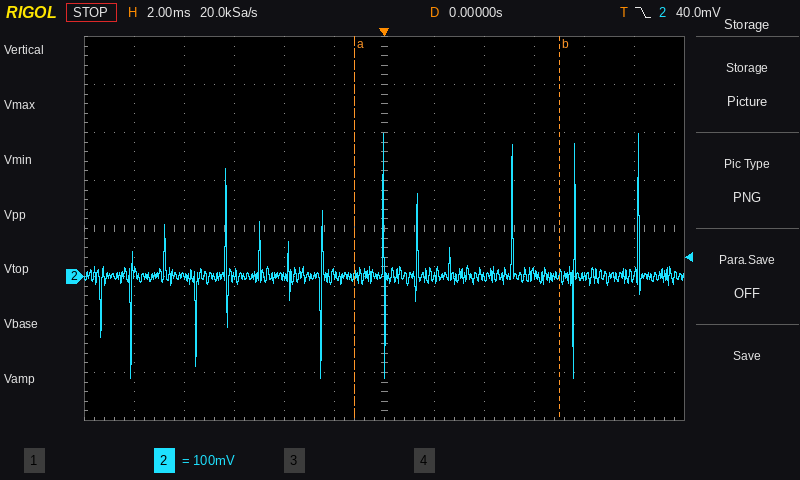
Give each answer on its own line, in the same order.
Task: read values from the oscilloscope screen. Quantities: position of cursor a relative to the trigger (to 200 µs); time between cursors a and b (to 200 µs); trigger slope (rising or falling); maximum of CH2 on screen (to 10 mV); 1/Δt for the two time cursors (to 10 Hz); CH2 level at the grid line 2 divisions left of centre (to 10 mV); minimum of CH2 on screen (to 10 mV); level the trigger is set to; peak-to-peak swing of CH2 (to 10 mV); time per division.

-1.2 ms
8.2 ms
falling
300 mV
120 Hz
0 mV
-210 mV
40.0 mV
510 mV
2 ms
